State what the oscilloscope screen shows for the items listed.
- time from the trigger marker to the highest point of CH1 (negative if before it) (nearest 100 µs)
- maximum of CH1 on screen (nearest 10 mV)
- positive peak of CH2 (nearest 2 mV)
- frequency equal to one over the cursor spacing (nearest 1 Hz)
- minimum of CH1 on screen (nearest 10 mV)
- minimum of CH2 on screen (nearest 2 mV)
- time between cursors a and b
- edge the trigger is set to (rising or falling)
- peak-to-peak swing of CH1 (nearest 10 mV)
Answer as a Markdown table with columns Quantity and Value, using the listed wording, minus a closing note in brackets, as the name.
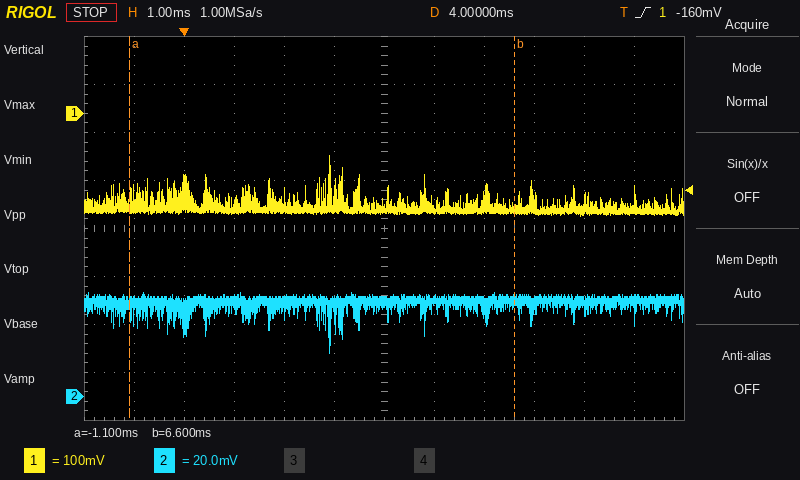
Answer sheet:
| Quantity | Value |
|---|---|
| time from the trigger marker to the highest point of CH1 (negative if before it) | +2.9 ms |
| maximum of CH1 on screen | -90 mV |
| positive peak of CH2 | 44 mV |
| frequency equal to one over the cursor spacing | 130 Hz |
| minimum of CH1 on screen | -210 mV |
| minimum of CH2 on screen | 18 mV |
| time between cursors a and b | 7.7 ms |
| edge the trigger is set to | rising |
| peak-to-peak swing of CH1 | 120 mV |
